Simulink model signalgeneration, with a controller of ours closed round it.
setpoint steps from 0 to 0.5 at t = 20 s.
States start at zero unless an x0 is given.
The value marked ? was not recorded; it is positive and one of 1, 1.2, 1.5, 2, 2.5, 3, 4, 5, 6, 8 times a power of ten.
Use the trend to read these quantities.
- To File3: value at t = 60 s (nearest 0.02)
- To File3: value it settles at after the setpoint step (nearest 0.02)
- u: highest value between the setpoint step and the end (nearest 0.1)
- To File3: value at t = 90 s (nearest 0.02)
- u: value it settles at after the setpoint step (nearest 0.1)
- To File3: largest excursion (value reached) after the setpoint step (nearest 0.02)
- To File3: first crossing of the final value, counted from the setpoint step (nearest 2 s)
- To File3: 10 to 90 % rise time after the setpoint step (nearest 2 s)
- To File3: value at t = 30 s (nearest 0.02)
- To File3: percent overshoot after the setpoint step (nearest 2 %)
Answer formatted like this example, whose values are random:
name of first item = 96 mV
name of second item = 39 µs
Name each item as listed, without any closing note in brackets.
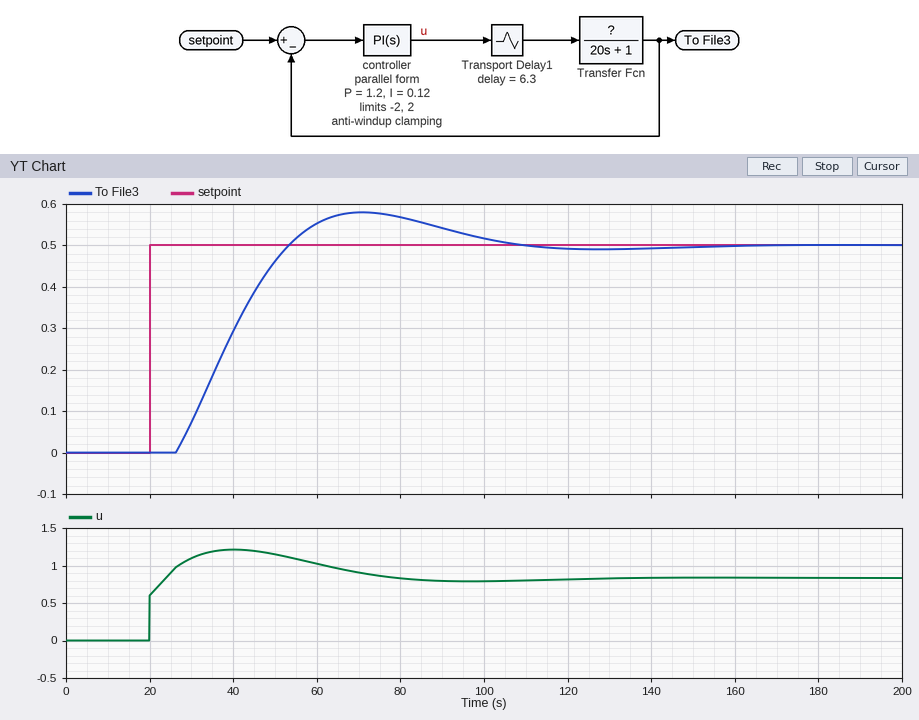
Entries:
To File3: value at t = 60 s = 0.56
To File3: value it settles at after the setpoint step = 0.50
u: highest value between the setpoint step and the end = 1.2
To File3: value at t = 90 s = 0.54
u: value it settles at after the setpoint step = 0.8
To File3: largest excursion (value reached) after the setpoint step = 0.58
To File3: first crossing of the final value, counted from the setpoint step = 34 s
To File3: 10 to 90 % rise time after the setpoint step = 20 s
To File3: value at t = 30 s = 0.08
To File3: percent overshoot after the setpoint step = 16 %
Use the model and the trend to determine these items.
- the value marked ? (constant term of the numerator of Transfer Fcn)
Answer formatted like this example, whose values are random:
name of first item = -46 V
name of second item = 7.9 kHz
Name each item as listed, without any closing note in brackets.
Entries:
the value marked ? = 0.6
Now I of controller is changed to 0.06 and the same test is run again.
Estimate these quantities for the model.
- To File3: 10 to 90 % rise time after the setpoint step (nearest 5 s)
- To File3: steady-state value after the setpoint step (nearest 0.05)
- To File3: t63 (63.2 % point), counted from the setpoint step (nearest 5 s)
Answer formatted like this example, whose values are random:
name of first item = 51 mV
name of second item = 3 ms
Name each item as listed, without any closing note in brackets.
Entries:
To File3: 10 to 90 % rise time after the setpoint step = 45 s
To File3: steady-state value after the setpoint step = 0.50
To File3: t63 (63.2 % point), counted from the setpoint step = 30 s
